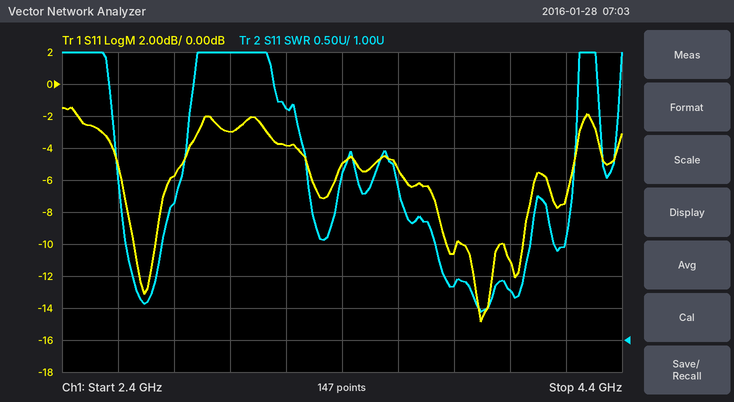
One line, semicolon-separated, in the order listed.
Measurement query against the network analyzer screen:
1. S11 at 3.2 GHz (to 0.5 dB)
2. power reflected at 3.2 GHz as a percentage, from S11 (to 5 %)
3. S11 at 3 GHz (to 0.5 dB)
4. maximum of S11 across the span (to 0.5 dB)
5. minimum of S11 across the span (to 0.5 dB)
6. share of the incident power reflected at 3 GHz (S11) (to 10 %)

-4.0 dB; 40 %; -3.0 dB; -1.5 dB; -15.0 dB; 50 %
